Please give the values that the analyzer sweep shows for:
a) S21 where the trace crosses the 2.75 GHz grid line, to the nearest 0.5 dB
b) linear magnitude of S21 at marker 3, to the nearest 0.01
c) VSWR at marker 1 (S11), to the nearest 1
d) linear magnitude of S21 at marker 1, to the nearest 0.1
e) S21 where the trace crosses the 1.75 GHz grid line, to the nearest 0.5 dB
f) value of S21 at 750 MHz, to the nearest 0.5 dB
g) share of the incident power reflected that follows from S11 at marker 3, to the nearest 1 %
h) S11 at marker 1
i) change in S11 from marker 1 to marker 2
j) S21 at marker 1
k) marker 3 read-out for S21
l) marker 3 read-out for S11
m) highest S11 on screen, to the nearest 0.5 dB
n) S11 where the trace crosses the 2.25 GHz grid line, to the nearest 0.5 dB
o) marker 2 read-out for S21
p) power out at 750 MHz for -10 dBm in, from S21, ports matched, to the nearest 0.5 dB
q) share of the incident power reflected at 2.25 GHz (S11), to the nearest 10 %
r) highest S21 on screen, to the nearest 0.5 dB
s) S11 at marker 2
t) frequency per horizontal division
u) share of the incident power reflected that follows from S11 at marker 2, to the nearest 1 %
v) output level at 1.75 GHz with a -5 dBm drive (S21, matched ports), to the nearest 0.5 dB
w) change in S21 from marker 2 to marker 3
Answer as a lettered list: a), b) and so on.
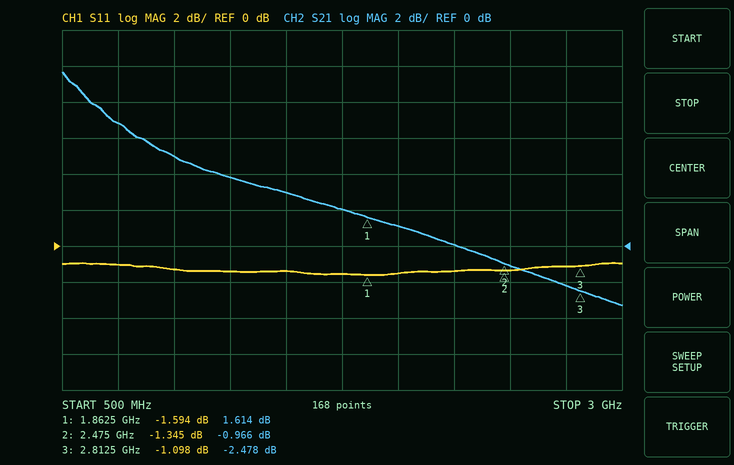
a) -2.0 dB
b) 0.75
c) 11
d) 1.2
e) 2.0 dB
f) 7.0 dB
g) 78 %
h) -1.594 dB
i) 0.249 dB
j) 1.614 dB
k) -2.478 dB
l) -1.098 dB
m) -1.0 dB
n) -1.5 dB
o) -0.966 dB
p) -3.0 dBm
q) 70 %
r) 9.5 dB
s) -1.345 dB
t) 250 MHz
u) 73 %
v) -3.0 dBm
w) -1.512 dB
